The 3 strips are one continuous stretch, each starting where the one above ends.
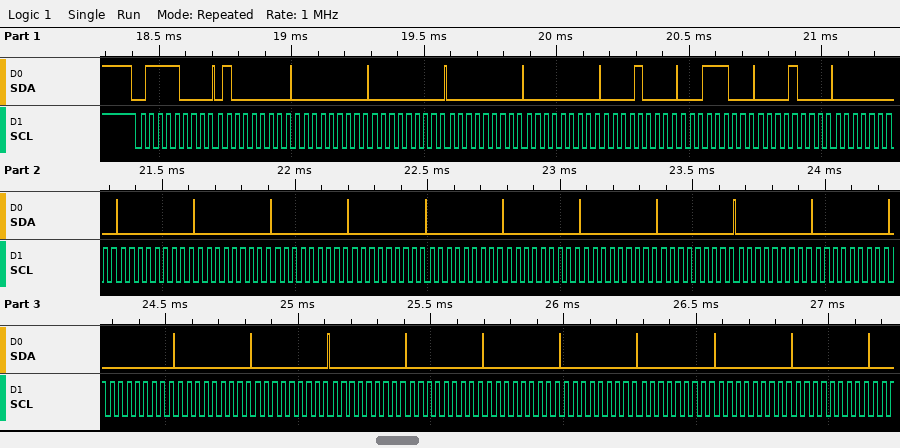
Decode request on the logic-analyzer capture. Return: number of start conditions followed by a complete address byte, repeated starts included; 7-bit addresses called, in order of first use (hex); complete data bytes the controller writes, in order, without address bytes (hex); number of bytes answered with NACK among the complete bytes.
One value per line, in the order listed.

1
0x3C
40 00 00 00 00 08 1C 08 00 00 00 00 00 00 00 00 00 00 00 00 00 00 00 00 00 00 00 00 00
0
